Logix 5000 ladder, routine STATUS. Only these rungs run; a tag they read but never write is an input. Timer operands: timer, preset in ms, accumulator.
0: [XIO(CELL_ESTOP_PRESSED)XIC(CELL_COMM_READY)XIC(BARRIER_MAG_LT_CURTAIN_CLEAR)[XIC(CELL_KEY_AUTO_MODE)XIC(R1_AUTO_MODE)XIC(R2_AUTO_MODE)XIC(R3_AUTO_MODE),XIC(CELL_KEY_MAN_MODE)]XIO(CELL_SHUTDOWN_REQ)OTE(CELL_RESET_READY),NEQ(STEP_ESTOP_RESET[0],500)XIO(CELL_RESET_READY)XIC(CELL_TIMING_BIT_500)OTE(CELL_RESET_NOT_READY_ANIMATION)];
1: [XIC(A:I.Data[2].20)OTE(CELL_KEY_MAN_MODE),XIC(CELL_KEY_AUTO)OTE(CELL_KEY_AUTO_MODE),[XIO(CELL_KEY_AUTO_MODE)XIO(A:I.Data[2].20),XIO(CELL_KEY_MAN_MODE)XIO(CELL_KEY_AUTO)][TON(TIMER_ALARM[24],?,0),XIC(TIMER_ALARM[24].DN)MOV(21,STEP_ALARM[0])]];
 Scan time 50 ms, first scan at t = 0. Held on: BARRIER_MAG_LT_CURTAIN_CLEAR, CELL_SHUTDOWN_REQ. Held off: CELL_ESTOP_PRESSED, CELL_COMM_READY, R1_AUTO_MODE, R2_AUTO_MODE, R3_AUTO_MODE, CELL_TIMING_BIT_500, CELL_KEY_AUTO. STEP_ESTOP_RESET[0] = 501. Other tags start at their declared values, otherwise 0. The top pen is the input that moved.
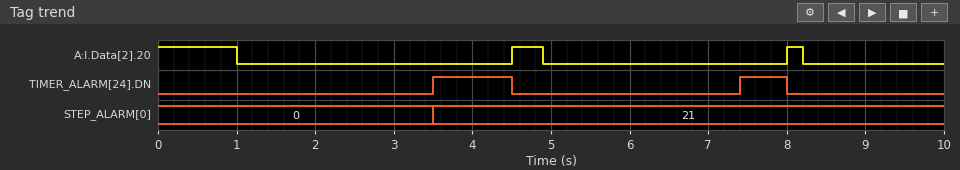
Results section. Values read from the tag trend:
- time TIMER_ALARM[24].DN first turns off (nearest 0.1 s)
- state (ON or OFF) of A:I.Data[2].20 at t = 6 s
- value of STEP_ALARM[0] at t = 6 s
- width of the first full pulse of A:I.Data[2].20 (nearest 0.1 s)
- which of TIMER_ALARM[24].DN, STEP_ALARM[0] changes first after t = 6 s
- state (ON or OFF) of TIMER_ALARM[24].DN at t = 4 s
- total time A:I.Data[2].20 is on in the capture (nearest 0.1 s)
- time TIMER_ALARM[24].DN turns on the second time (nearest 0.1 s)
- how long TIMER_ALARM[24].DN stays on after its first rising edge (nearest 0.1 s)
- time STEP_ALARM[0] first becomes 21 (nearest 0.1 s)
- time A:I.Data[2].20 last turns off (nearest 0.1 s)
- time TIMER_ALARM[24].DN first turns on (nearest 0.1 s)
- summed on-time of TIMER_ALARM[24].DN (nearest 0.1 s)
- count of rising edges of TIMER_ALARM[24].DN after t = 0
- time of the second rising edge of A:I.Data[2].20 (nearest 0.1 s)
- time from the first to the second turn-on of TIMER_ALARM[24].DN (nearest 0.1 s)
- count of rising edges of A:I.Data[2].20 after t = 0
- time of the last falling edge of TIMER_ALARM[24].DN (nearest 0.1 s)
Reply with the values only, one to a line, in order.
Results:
4.5 s
OFF
21
0.4 s
TIMER_ALARM[24].DN
ON
1.6 s
7.4 s
1.0 s
3.5 s
8.2 s
3.5 s
1.6 s
2
8.0 s
3.9 s
2
8.0 s
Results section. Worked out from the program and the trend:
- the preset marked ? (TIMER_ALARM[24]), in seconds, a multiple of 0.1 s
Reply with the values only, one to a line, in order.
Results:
2.5 s
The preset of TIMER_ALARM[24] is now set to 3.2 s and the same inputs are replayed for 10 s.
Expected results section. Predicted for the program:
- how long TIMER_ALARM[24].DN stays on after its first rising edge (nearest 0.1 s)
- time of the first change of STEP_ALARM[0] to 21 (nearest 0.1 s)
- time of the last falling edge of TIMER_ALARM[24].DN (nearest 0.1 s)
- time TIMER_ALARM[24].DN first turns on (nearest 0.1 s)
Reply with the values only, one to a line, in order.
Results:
0.3 s
4.2 s
4.5 s
4.2 s
